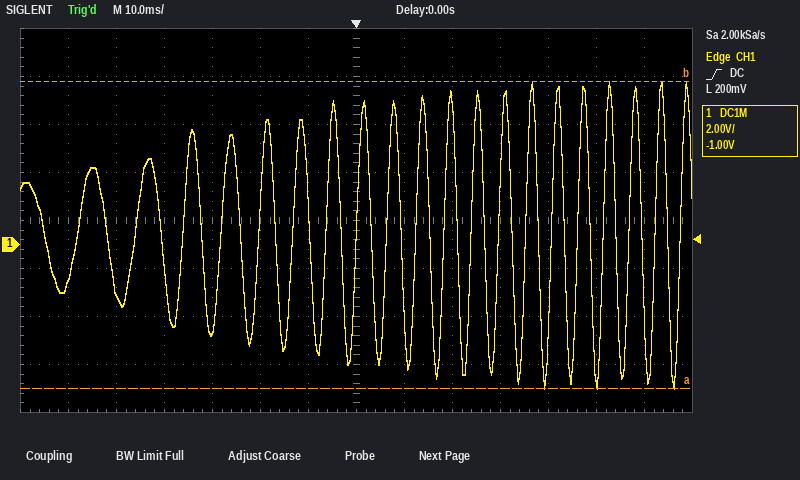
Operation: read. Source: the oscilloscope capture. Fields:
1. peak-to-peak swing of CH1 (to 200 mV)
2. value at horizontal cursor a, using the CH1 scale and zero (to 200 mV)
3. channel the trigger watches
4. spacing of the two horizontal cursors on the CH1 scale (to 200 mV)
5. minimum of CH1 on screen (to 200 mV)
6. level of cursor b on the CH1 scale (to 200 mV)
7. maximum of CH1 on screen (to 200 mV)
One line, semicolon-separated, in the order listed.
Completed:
12.8 V; -6.0 V; CH1; 12.8 V; -6.0 V; 6.8 V; 6.8 V
